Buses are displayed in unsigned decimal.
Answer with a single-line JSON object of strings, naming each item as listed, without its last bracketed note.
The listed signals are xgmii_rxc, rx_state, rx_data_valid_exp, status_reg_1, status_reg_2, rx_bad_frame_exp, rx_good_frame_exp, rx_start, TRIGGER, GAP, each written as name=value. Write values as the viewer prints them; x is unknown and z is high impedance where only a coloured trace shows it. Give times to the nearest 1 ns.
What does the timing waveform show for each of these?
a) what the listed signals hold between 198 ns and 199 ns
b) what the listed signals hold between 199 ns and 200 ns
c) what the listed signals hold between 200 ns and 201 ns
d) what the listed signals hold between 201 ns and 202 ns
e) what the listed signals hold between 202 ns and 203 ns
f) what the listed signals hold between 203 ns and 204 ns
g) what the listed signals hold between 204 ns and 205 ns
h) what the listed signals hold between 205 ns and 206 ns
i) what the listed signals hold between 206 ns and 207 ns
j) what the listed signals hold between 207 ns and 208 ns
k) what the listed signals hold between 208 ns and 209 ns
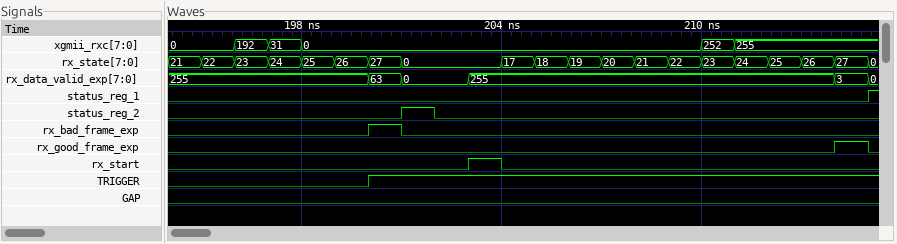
{"what the listed signals hold between 198 ns and 199 ns": "xgmii_rxc=0, rx_state=25, rx_data_valid_exp=255, status_reg_1=0, status_reg_2=0, rx_bad_frame_exp=0, rx_good_frame_exp=0, rx_start=0, TRIGGER=0, GAP=0", "what the listed signals hold between 199 ns and 200 ns": "xgmii_rxc=0, rx_state=26, rx_data_valid_exp=255, status_reg_1=0, status_reg_2=0, rx_bad_frame_exp=0, rx_good_frame_exp=0, rx_start=0, TRIGGER=0, GAP=0", "what the listed signals hold between 200 ns and 201 ns": "xgmii_rxc=0, rx_state=27, rx_data_valid_exp=63, status_reg_1=0, status_reg_2=0, rx_bad_frame_exp=1, rx_good_frame_exp=0, rx_start=0, TRIGGER=1, GAP=0", "what the listed signals hold between 201 ns and 202 ns": "xgmii_rxc=0, rx_state=0, rx_data_valid_exp=0, status_reg_1=0, status_reg_2=1, rx_bad_frame_exp=0, rx_good_frame_exp=0, rx_start=0, TRIGGER=1, GAP=0", "what the listed signals hold between 202 ns and 203 ns": "xgmii_rxc=0, rx_state=0, rx_data_valid_exp=0, status_reg_1=0, status_reg_2=0, rx_bad_frame_exp=0, rx_good_frame_exp=0, rx_start=0, TRIGGER=1, GAP=0", "what the listed signals hold between 203 ns and 204 ns": "xgmii_rxc=0, rx_state=0, rx_data_valid_exp=255, status_reg_1=0, status_reg_2=0, rx_bad_frame_exp=0, rx_good_frame_exp=0, rx_start=1, TRIGGER=1, GAP=0", "what the listed signals hold between 204 ns and 205 ns": "xgmii_rxc=0, rx_state=17, rx_data_valid_exp=255, status_reg_1=0, status_reg_2=0, rx_bad_frame_exp=0, rx_good_frame_exp=0, rx_start=0, TRIGGER=1, GAP=0", "what the listed signals hold between 205 ns and 206 ns": "xgmii_rxc=0, rx_state=18, rx_data_valid_exp=255, status_reg_1=0, status_reg_2=0, rx_bad_frame_exp=0, rx_good_frame_exp=0, rx_start=0, TRIGGER=1, GAP=0", "what the listed signals hold between 206 ns and 207 ns": "xgmii_rxc=0, rx_state=19, rx_data_valid_exp=255, status_reg_1=0, status_reg_2=0, rx_bad_frame_exp=0, rx_good_frame_exp=0, rx_start=0, TRIGGER=1, GAP=0", "what the listed signals hold between 207 ns and 208 ns": "xgmii_rxc=0, rx_state=20, rx_data_valid_exp=255, status_reg_1=0, status_reg_2=0, rx_bad_frame_exp=0, rx_good_frame_exp=0, rx_start=0, TRIGGER=1, GAP=0", "what the listed signals hold between 208 ns and 209 ns": "xgmii_rxc=0, rx_state=21, rx_data_valid_exp=255, status_reg_1=0, status_reg_2=0, rx_bad_frame_exp=0, rx_good_frame_exp=0, rx_start=0, TRIGGER=1, GAP=0"}
